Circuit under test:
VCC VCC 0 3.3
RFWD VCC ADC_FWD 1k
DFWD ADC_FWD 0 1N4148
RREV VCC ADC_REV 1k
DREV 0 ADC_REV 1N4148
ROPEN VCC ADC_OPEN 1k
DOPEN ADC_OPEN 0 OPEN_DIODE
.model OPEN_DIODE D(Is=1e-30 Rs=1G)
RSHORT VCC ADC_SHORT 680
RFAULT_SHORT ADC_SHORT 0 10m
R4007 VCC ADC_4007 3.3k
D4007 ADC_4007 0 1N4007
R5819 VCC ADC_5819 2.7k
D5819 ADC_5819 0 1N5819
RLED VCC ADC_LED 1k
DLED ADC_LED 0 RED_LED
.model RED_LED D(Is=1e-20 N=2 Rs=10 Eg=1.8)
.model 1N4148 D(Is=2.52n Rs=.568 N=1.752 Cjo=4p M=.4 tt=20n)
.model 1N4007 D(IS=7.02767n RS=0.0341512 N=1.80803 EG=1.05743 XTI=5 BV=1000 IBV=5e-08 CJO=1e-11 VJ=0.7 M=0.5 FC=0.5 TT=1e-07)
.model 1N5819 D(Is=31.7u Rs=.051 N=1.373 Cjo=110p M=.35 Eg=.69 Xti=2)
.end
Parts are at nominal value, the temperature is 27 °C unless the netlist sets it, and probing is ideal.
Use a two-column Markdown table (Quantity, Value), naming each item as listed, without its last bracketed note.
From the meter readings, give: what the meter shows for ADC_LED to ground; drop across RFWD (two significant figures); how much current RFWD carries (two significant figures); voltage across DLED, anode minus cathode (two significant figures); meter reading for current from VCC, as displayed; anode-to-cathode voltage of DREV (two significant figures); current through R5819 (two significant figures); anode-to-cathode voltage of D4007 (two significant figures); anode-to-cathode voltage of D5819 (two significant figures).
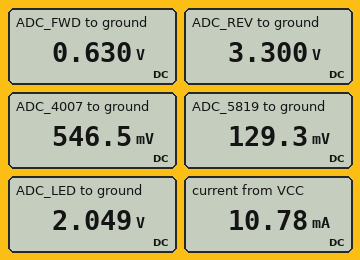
| Quantity | Value |
|---|---|
| what the meter shows for ADC_LED to ground | 2.049 V |
| drop across RFWD | 2.7 V |
| how much current RFWD carries | 2.7 mA |
| voltage across DLED, anode minus cathode | 2.0 V |
| meter reading for current from VCC, as displayed | 10.78 mA |
| anode-to-cathode voltage of DREV | -3.3 V |
| current through R5819 | 1.2 mA |
| anode-to-cathode voltage of D4007 | 550 mV |
| anode-to-cathode voltage of D5819 | 130 mV |
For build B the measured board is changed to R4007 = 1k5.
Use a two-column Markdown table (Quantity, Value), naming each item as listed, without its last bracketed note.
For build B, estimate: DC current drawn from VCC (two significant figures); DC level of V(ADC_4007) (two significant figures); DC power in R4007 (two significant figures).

| Quantity | Value |
|---|---|
| DC current drawn from VCC | 12 mA |
| DC level of V(ADC_4007) | 580 mV |
| DC power in R4007 | 4.9 mW |
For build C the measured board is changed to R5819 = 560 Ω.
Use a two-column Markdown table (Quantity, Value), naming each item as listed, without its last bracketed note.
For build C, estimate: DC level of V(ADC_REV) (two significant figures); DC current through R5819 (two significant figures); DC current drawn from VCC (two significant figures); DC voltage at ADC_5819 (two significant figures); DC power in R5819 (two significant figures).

| Quantity | Value |
|---|---|
| DC level of V(ADC_REV) | 3.3 V |
| DC current through R5819 | 5.6 mA |
| DC current drawn from VCC | 15 mA |
| DC voltage at ADC_5819 | 180 mV |
| DC power in R5819 | 17 mW |
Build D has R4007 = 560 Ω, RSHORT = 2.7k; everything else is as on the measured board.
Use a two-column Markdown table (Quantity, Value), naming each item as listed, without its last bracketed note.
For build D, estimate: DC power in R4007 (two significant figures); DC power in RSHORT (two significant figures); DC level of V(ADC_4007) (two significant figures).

| Quantity | Value |
|---|---|
| DC power in R4007 | 13 mW |
| DC power in RSHORT | 4.0 mW |
| DC level of V(ADC_4007) | 630 mV |
